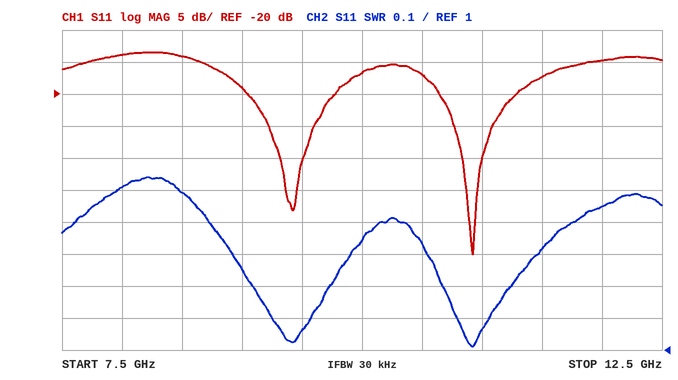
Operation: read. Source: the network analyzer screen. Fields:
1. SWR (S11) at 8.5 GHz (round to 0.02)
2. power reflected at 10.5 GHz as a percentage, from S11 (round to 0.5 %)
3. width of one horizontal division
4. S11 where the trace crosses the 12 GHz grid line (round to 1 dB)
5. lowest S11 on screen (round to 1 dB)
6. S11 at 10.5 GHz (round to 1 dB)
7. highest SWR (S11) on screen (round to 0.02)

1.50
2.0 %
500 MHz
-15 dB
-45 dB
-17 dB
1.54
